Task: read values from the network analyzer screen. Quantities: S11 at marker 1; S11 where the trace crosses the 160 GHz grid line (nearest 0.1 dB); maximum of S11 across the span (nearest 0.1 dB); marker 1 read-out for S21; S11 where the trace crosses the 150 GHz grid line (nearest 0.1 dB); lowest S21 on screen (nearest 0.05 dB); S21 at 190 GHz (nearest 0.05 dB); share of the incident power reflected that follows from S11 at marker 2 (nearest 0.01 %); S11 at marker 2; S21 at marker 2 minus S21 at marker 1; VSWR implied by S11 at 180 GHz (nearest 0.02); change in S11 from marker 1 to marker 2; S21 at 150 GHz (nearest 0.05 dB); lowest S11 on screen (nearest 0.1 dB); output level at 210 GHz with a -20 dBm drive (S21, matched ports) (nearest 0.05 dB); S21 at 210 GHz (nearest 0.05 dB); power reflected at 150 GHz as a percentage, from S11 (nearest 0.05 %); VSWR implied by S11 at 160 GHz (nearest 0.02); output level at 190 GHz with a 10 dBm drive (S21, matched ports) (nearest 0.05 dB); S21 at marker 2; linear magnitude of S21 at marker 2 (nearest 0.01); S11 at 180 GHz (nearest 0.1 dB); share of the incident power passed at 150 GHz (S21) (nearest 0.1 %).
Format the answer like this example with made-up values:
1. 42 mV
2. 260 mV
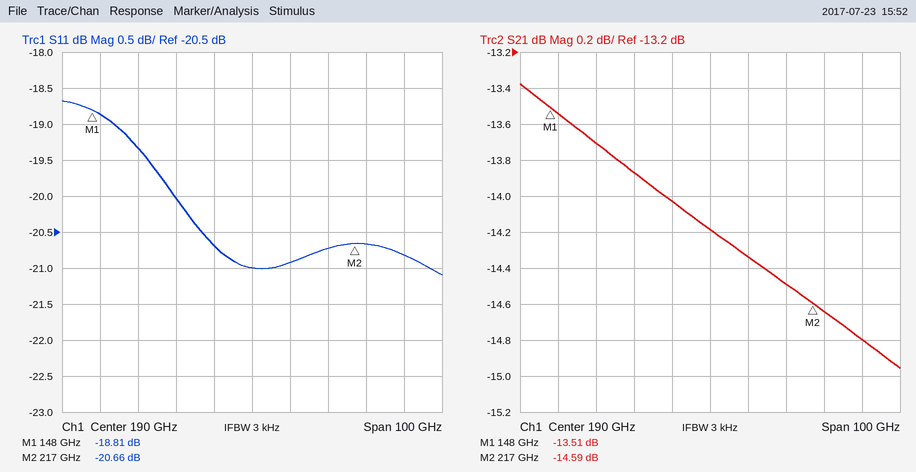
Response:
1. -18.81 dB
2. -19.3 dB
3. -18.7 dB
4. -13.51 dB
5. -18.9 dB
6. -14.95 dB
7. -14.20 dB
8. 0.86 %
9. -20.66 dB
10. -1.08 dB
11. 1.20
12. -1.85 dB
13. -13.55 dB
14. -21.1 dB
15. -34.50 dBm
16. -14.50 dB
17. 1.30 %
18. 1.24
19. -4.20 dBm
20. -14.59 dB
21. 0.19
22. -20.7 dB
23. 4.4 %
